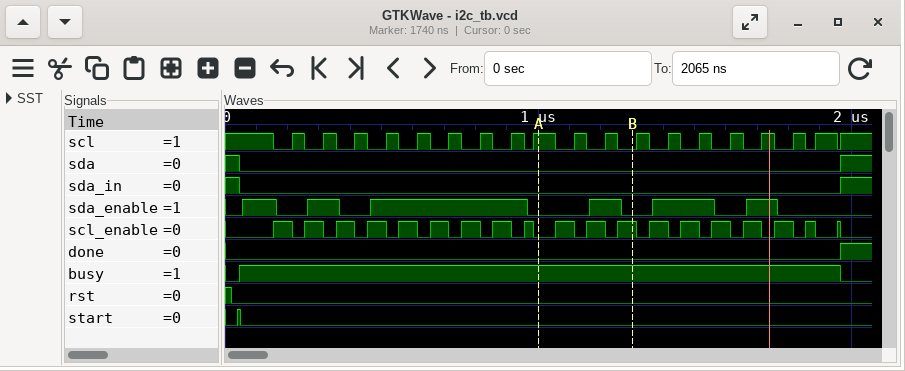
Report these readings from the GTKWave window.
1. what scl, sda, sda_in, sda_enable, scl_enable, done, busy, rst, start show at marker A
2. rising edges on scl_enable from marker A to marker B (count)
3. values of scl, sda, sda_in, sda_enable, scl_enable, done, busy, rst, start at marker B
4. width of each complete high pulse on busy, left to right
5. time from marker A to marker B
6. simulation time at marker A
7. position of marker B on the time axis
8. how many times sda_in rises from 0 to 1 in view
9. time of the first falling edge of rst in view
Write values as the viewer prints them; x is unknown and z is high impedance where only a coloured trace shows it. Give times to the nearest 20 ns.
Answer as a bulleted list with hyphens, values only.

- scl=1, sda=0, sda_in=0, sda_enable=0, scl_enable=0, done=0, busy=1, rst=0, start=0
- 3
- scl=0, sda=0, sda_in=0, sda_enable=0, scl_enable=1, done=0, busy=1, rst=0, start=0
- 1920 ns
- 300 ns
- 1000 ns
- 1300 ns
- 1
- 20 ns
